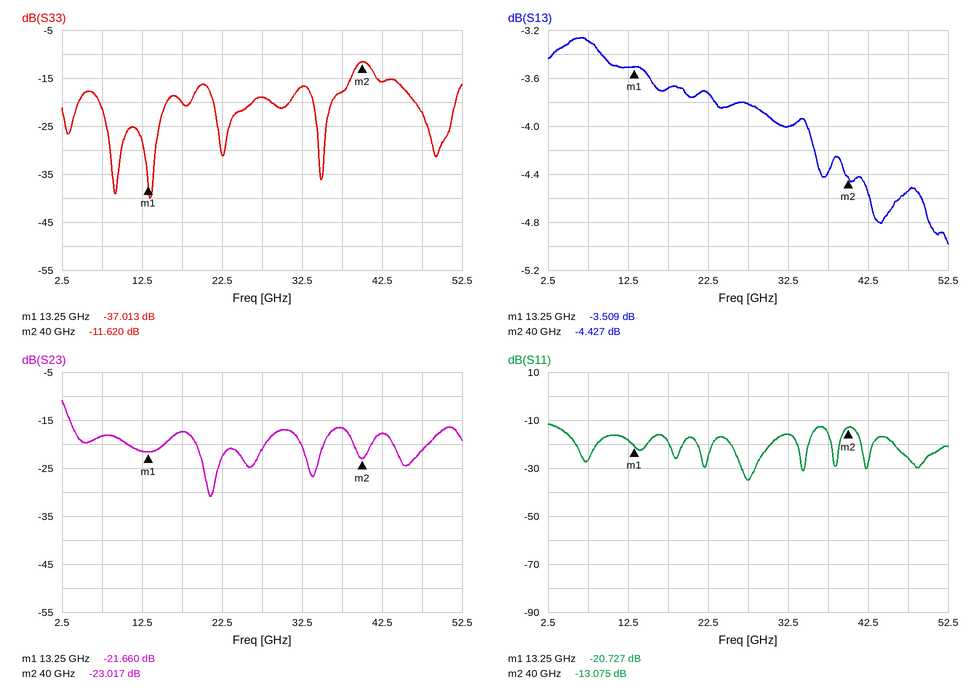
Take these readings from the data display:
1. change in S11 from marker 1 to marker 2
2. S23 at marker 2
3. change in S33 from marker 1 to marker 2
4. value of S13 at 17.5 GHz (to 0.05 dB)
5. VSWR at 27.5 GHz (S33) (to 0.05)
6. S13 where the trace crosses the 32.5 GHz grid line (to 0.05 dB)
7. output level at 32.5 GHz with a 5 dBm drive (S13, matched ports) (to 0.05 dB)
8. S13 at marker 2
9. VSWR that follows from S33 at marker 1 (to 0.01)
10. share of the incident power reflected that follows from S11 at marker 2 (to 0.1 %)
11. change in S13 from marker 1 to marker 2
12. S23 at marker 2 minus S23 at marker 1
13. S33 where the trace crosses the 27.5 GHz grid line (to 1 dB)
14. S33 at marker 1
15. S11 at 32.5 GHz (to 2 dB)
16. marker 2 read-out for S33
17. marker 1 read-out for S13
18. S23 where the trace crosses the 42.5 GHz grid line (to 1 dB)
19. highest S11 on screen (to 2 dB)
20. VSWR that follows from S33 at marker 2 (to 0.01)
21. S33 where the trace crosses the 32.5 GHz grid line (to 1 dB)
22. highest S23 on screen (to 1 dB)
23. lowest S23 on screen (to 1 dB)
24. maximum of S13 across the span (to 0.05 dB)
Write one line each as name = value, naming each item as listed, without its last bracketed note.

change in S11 from marker 1 to marker 2 = 7.652 dB
S23 at marker 2 = -23.017 dB
change in S33 from marker 1 to marker 2 = 25.393 dB
value of S13 at 17.5 GHz = -3.70 dB
VSWR at 27.5 GHz (S33) = 1.25
S13 where the trace crosses the 32.5 GHz grid line = -4.00 dB
output level at 32.5 GHz with a 5 dBm drive (S13, matched ports) = 1.00 dBm
S13 at marker 2 = -4.427 dB
VSWR that follows from S33 at marker 1 = 1.03
share of the incident power reflected that follows from S11 at marker 2 = 4.9 %
change in S13 from marker 1 to marker 2 = -0.918 dB
S23 at marker 2 minus S23 at marker 1 = -1.357 dB
S33 where the trace crosses the 27.5 GHz grid line = -19 dB
S33 at marker 1 = -37.013 dB
S11 at 32.5 GHz = -16 dB
marker 2 read-out for S33 = -11.620 dB
marker 1 read-out for S13 = -3.509 dB
S23 where the trace crosses the 42.5 GHz grid line = -18 dB
highest S11 on screen = -12 dB
VSWR that follows from S33 at marker 2 = 1.71
S33 where the trace crosses the 32.5 GHz grid line = -17 dB
highest S23 on screen = -11 dB
lowest S23 on screen = -31 dB
maximum of S13 across the span = -3.25 dB
